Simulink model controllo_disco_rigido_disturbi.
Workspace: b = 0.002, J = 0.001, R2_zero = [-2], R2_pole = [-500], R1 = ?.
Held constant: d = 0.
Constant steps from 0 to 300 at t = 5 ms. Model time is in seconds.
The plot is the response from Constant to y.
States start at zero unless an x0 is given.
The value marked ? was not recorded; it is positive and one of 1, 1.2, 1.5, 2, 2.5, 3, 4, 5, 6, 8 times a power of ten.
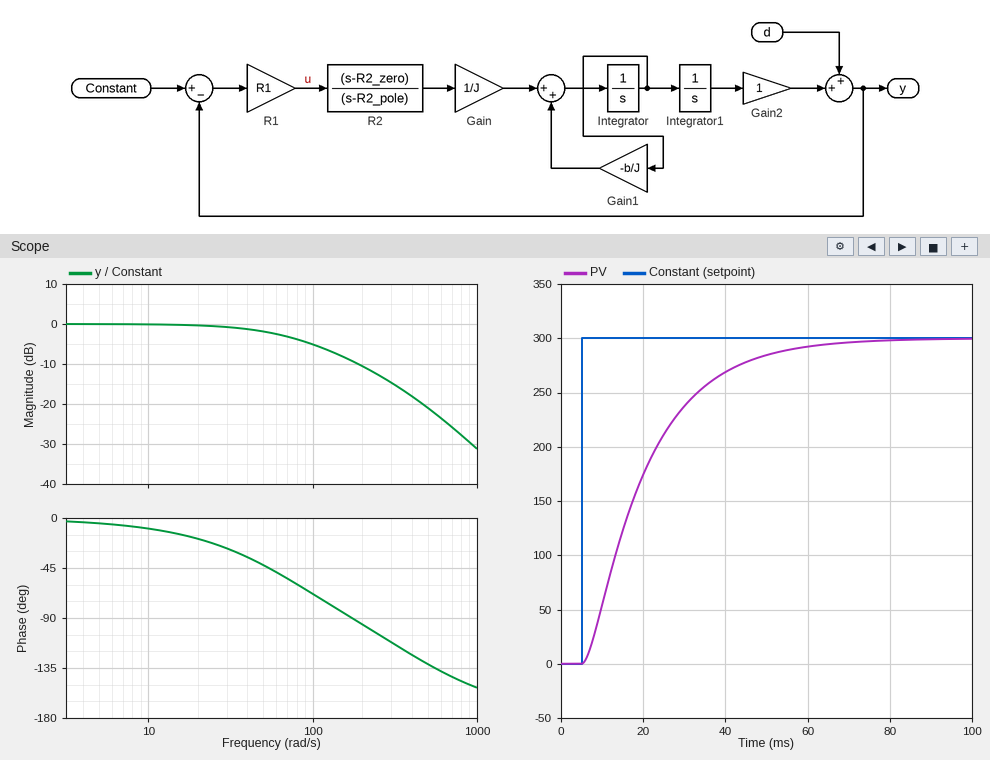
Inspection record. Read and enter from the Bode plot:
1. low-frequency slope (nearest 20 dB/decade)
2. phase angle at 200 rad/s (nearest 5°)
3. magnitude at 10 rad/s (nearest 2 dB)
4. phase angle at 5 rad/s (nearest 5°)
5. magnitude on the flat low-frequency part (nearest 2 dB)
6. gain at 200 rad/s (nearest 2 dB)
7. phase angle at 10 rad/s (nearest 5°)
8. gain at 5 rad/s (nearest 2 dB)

0 dB/decade
-95°
0 dB
-5°
0 dB
-10 dB
-10°
0 dB
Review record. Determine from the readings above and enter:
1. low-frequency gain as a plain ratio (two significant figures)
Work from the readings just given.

1.0
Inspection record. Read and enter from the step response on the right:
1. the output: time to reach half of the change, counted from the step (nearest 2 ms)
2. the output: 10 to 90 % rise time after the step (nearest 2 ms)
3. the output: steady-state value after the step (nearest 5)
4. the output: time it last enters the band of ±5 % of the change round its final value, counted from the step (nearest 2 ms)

12 ms
32 ms
300
46 ms
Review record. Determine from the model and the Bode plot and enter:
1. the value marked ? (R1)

30
